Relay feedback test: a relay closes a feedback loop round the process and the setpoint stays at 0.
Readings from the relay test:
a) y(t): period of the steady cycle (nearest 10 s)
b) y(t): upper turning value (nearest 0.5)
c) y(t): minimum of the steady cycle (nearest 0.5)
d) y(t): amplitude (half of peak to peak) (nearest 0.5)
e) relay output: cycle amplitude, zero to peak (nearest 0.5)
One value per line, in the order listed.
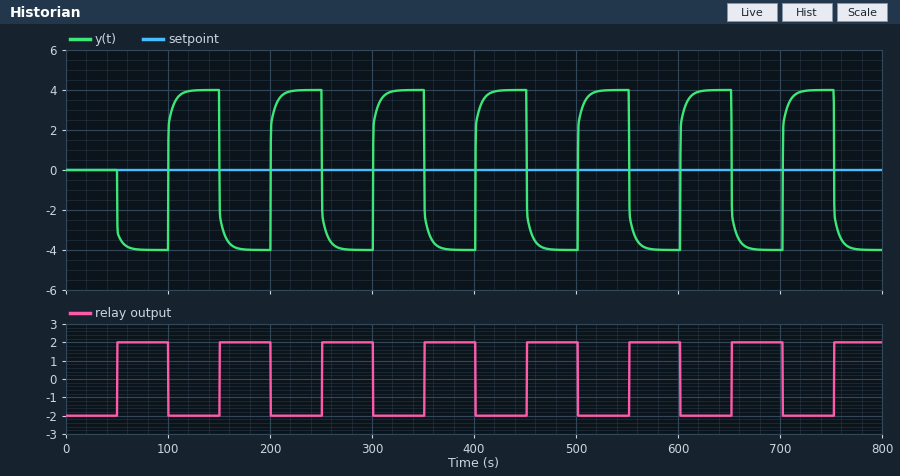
100 s
4.0
-4.0
4.0
2.0
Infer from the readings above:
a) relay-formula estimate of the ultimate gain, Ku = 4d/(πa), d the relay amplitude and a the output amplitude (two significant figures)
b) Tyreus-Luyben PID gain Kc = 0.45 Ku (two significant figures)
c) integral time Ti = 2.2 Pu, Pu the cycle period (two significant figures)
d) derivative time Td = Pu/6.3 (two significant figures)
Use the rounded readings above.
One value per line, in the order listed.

0.64
0.29
220 s
16 s
